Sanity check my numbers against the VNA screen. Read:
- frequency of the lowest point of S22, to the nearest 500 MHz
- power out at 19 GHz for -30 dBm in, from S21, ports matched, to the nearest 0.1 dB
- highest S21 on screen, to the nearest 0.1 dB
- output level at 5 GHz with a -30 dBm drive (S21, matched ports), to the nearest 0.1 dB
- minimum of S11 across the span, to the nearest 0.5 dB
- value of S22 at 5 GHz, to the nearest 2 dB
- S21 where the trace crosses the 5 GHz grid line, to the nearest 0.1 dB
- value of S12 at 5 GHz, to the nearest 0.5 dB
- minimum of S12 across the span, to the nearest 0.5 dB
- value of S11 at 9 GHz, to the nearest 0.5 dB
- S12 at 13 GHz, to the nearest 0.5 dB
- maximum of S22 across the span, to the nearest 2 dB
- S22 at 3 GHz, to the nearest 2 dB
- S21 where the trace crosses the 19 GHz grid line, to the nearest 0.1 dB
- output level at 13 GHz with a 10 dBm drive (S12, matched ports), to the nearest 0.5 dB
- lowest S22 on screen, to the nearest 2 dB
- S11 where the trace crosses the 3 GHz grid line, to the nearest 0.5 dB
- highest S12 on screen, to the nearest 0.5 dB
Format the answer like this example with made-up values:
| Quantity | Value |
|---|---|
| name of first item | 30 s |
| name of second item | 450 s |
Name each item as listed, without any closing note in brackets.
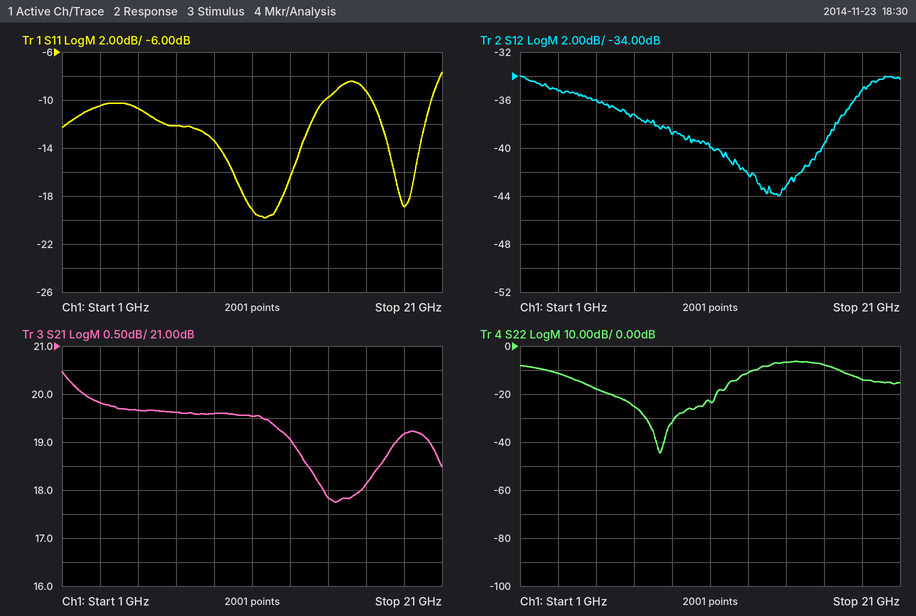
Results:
| Quantity | Value |
|---|---|
| frequency of the lowest point of S22, to the nearest 500 MHz | 8.5 GHz |
| power out at 19 GHz for -30 dBm in, from S21, ports matched, to the nearest 0.1 dB | -10.8 dBm |
| highest S21 on screen, to the nearest 0.1 dB | 20.5 dB |
| output level at 5 GHz with a -30 dBm drive (S21, matched ports), to the nearest 0.1 dB | -10.3 dBm |
| minimum of S11 across the span, to the nearest 0.5 dB | -20.0 dB |
| value of S22 at 5 GHz, to the nearest 2 dB | -18 dB |
| S21 where the trace crosses the 5 GHz grid line, to the nearest 0.1 dB | 19.7 dB |
| value of S12 at 5 GHz, to the nearest 0.5 dB | -36.0 dB |
| minimum of S12 across the span, to the nearest 0.5 dB | -44.0 dB |
| value of S11 at 9 GHz, to the nearest 0.5 dB | -13.5 dB |
| S12 at 13 GHz, to the nearest 0.5 dB | -42.0 dB |
| maximum of S22 across the span, to the nearest 2 dB | -6 dB |
| S22 at 3 GHz, to the nearest 2 dB | -12 dB |
| S21 where the trace crosses the 19 GHz grid line, to the nearest 0.1 dB | 19.2 dB |
| output level at 13 GHz with a 10 dBm drive (S12, matched ports), to the nearest 0.5 dB | -32.0 dBm |
| lowest S22 on screen, to the nearest 2 dB | -44 dB |
| S11 where the trace crosses the 3 GHz grid line, to the nearest 0.5 dB | -10.5 dB |
| highest S12 on screen, to the nearest 0.5 dB | -34.0 dB |
